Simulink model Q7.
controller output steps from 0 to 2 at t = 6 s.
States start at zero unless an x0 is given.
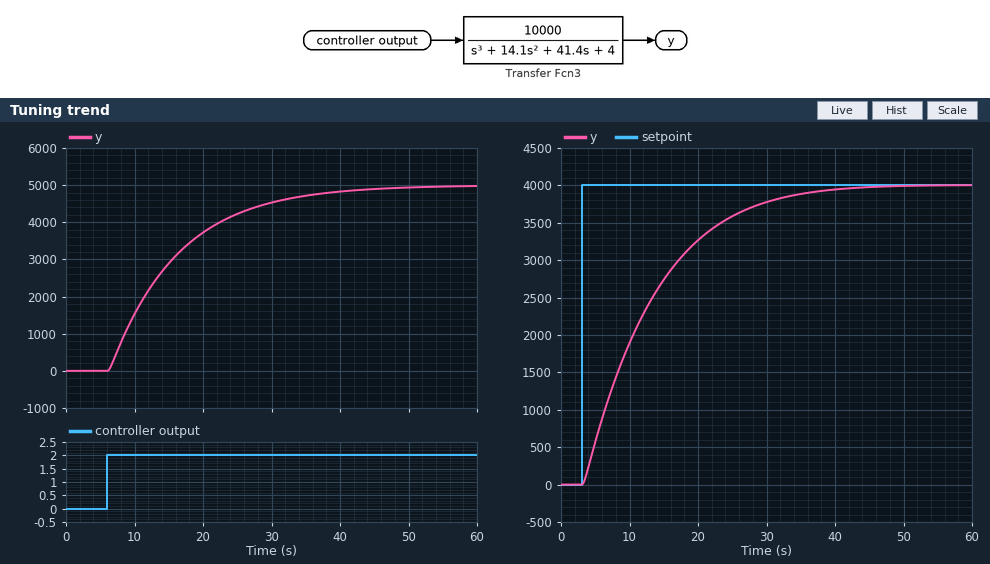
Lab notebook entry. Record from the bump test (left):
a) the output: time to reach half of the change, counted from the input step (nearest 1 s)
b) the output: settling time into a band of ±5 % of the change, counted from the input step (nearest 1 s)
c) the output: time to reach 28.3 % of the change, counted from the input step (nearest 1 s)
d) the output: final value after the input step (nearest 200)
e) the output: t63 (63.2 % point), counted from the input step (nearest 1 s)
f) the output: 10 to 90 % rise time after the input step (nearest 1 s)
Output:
7 s
30 s
4 s
5000
10 s
22 s
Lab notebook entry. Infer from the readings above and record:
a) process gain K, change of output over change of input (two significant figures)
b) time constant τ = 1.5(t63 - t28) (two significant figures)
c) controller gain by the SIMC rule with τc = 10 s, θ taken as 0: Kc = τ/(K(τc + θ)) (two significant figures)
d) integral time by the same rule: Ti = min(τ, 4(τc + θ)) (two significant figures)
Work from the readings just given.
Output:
2500
9.0 s
0.00036
9.0 s
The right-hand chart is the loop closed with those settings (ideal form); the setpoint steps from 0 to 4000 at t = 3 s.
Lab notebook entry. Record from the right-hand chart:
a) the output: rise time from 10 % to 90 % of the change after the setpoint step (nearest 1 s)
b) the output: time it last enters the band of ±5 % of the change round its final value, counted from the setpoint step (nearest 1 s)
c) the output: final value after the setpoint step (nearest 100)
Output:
21 s
28 s
4000
